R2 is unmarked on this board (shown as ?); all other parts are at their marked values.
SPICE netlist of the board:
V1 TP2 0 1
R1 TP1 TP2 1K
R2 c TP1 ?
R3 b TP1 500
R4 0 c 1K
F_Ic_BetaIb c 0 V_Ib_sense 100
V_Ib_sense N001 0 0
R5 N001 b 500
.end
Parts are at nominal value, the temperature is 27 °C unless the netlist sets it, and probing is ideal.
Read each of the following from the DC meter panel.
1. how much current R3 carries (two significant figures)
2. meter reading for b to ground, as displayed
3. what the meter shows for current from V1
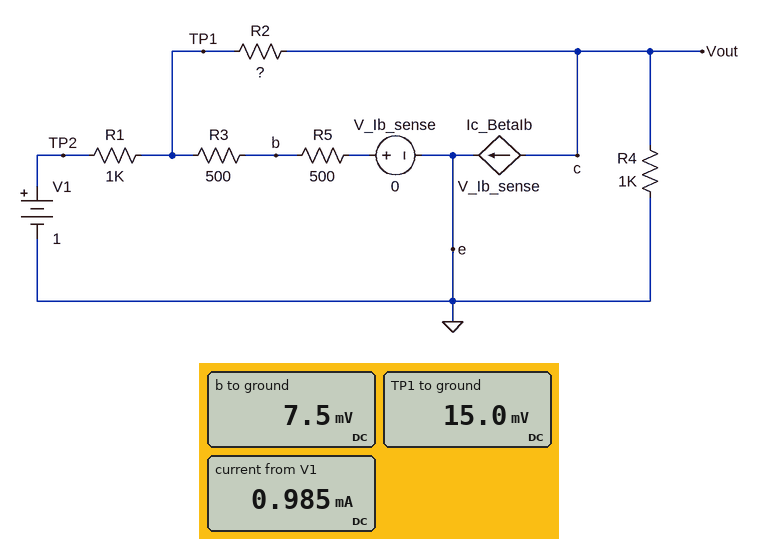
15 µA
7.5 mV
0.985 mA
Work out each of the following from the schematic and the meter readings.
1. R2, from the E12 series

560 Ω
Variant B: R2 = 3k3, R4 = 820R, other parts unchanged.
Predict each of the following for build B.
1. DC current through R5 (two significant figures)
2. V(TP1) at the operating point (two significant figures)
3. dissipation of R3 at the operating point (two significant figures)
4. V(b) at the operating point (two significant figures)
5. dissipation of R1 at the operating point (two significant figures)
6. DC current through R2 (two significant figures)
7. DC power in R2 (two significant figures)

45 µA
45 mV
1.0 µW
23 mV
910 µW
910 µA
2.7 mW
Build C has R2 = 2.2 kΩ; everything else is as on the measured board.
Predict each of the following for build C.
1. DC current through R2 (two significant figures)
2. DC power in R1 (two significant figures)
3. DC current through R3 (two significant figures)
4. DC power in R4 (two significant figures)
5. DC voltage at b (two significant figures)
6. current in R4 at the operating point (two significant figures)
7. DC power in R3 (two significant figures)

940 µA
940 µW
30 µA
4.2 mW
15 mV
2.0 mA
440 nW
